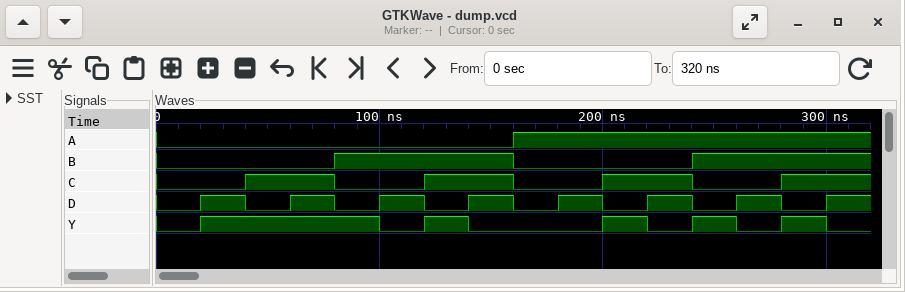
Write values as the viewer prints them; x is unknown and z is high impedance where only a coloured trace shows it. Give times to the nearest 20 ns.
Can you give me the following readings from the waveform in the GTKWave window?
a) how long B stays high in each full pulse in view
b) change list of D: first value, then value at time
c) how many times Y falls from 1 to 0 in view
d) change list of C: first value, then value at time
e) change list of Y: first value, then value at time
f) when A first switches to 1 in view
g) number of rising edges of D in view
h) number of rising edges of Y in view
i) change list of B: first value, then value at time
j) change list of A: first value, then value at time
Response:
80 ns
0, 1 at 20 ns, 0 at 40 ns, 1 at 60 ns, 0 at 80 ns, 1 at 100 ns, 0 at 120 ns, 1 at 140 ns, 0 at 160 ns, 1 at 180 ns, 0 at 200 ns, 1 at 220 ns, 0 at 240 ns, 1 at 260 ns, 0 at 280 ns, 1 at 300 ns
5
0, 1 at 40 ns, 0 at 80 ns, 1 at 120 ns, 0 at 160 ns, 1 at 200 ns, 0 at 240 ns, 1 at 280 ns
0, 1 at 20 ns, 0 at 100 ns, 1 at 120 ns, 0 at 140 ns, 1 at 200 ns, 0 at 220 ns, 1 at 240 ns, 0 at 260 ns, 1 at 280 ns, 0 at 300 ns
160 ns
8
5
0, 1 at 80 ns, 0 at 160 ns, 1 at 240 ns
0, 1 at 160 ns
